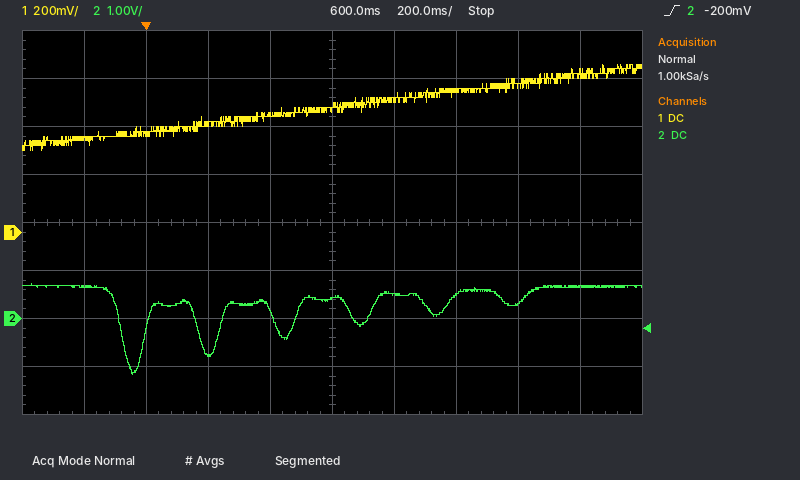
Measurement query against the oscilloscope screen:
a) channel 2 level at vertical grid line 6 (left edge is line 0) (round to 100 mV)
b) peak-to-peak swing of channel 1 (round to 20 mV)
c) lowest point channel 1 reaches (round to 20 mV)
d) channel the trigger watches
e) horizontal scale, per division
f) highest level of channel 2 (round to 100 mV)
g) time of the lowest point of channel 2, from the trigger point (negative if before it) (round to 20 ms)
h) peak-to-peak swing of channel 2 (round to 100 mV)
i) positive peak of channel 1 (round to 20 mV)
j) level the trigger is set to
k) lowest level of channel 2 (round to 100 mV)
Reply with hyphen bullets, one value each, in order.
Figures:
- 500 mV
- 360 mV
- 340 mV
- channel 2
- 200 ms
- 700 mV
- -40 ms
- 1.9 V
- 700 mV
- -200 mV
- -1.2 V
